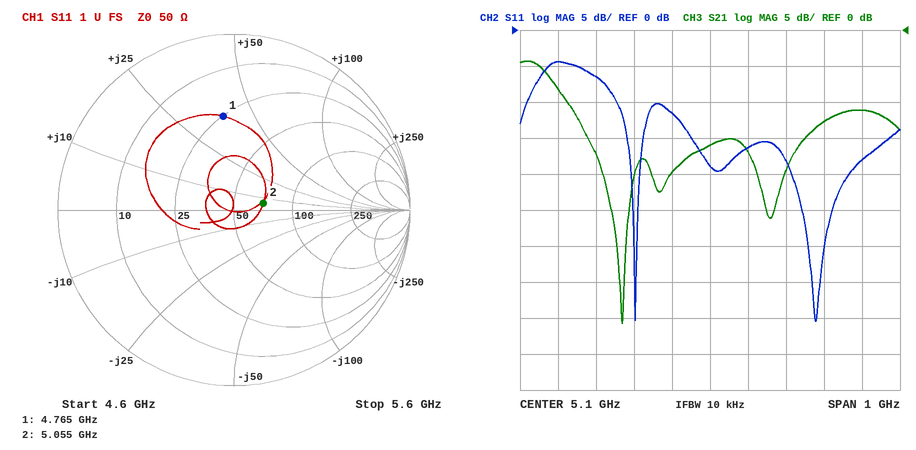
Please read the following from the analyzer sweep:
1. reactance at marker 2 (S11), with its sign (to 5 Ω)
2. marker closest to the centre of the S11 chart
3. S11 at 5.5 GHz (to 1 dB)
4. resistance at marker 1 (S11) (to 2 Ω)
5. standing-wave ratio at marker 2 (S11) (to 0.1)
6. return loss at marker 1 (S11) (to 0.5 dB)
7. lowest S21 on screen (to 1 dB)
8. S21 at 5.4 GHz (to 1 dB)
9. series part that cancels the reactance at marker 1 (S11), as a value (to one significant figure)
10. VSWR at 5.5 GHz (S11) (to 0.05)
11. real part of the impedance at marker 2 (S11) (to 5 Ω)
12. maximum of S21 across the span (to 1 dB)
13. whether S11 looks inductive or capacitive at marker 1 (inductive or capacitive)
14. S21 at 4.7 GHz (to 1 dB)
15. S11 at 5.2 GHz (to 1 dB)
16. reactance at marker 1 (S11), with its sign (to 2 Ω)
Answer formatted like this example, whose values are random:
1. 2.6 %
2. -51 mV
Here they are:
1. +5 Ω
2. marker 2
3. -18 dB
4. 26 Ω
5. 1.4
6. 5.5 dB
7. -41 dB
8. -13 dB
9. 900 fF
10. 1.30
11. 70 Ω
12. -4 dB
13. inductive
14. -8 dB
15. -16 dB
16. +38 Ω
